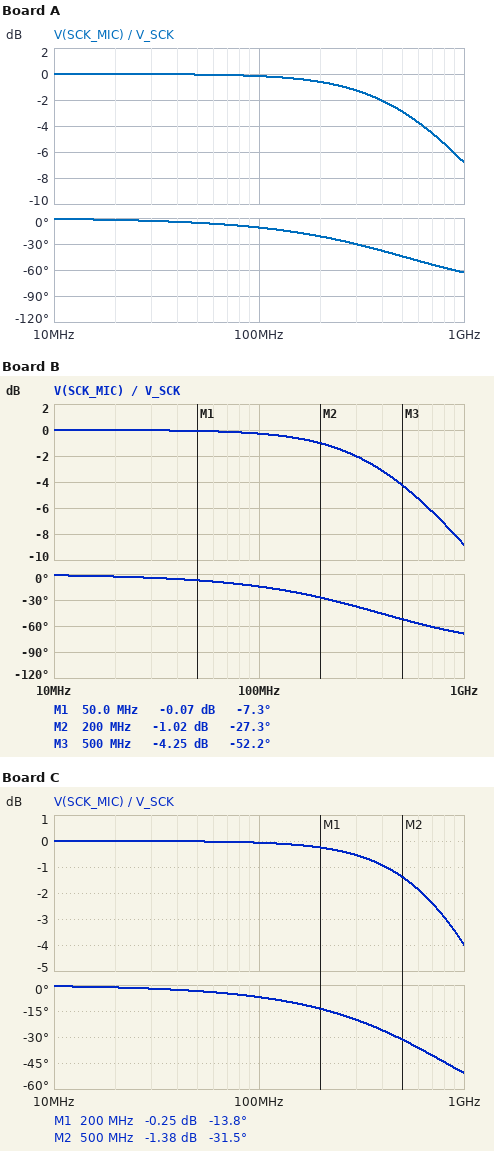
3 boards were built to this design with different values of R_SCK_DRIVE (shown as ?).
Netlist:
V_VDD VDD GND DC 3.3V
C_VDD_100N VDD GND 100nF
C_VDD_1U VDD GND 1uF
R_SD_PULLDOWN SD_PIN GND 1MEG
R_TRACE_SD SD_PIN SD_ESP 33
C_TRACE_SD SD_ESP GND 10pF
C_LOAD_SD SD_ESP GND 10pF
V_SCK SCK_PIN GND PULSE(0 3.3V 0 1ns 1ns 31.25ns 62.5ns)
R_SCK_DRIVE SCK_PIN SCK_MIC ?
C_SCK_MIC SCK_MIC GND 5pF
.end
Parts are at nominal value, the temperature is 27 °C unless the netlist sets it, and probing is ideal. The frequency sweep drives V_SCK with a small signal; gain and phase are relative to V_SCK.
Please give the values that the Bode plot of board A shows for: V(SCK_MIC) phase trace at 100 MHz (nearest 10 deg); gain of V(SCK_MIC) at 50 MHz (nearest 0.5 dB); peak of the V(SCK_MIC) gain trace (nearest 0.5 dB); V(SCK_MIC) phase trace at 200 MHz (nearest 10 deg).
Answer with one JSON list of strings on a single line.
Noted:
["-10 deg", "0 dB", "0 dB", "-20 deg"]
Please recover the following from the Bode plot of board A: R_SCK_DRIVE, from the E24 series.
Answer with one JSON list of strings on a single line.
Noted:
["62 Ω"]
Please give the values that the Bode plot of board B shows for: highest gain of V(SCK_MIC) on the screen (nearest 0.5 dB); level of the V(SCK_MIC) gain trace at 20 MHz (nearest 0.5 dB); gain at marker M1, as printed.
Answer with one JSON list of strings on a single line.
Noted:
["0 dB", "0 dB", "-0.07 dB"]
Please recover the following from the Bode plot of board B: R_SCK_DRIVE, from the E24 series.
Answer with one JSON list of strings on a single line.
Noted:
["82 Ω"]
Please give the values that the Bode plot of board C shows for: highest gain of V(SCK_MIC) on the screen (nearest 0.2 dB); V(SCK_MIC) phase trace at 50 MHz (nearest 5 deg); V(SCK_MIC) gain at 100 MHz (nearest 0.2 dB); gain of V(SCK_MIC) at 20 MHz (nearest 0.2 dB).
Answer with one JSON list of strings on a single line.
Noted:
["0 dB", "-5 deg", "0 dB", "0 dB"]
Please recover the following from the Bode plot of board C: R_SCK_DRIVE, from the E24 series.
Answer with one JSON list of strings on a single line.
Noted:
["39 Ω"]
